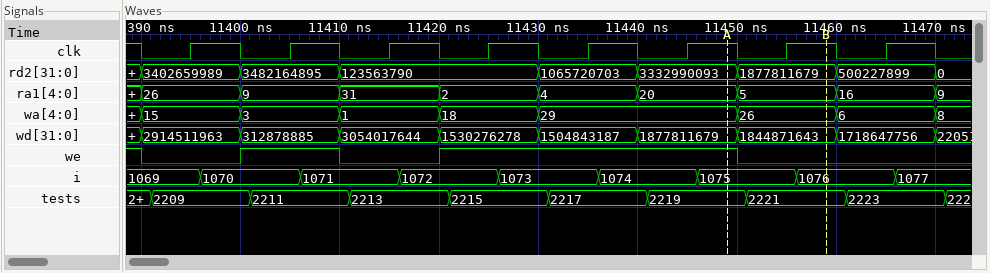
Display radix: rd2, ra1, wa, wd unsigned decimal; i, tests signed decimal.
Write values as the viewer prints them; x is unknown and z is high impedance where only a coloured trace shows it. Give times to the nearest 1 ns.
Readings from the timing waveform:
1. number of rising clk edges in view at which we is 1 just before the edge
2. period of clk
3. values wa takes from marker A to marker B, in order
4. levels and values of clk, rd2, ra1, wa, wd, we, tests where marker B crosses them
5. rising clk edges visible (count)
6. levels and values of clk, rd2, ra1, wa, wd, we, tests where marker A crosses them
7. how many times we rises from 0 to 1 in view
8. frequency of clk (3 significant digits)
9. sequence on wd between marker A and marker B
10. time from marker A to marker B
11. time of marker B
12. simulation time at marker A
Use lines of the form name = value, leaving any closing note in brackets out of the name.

number of rising clk edges in view at which we is 1 just before the edge = 4
period of clk = 10 ns
values wa takes from marker A to marker B, in order = 29, 26
levels and values of clk, rd2, ra1, wa, wd, we, tests where marker B crosses them = clk=1, rd2=1877811679, ra1=5, wa=26, wd=1844871643, we=0, tests=2221
rising clk edges visible = 8
levels and values of clk, rd2, ra1, wa, wd, we, tests where marker A crosses them = clk=1, rd2=3332990093, ra1=20, wa=29, wd=1877811679, we=1, tests=2219
how many times we rises from 0 to 1 in view = 2
frequency of clk = 100 MHz
sequence on wd between marker A and marker B = 1877811679, 1844871643
time from marker A to marker B = 10 ns
time of marker B = 11459 ns
simulation time at marker A = 11449 ns
